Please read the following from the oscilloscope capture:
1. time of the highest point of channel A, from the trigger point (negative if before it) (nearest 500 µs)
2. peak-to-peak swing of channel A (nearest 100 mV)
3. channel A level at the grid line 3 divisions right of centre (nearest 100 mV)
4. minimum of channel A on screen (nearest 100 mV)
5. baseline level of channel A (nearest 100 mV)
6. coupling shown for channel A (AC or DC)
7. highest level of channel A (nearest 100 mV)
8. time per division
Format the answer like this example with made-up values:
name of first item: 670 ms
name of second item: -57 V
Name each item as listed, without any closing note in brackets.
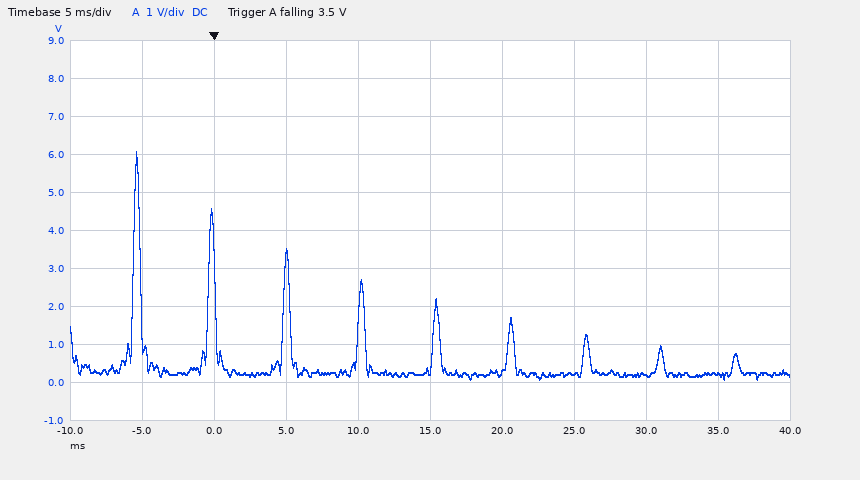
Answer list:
time of the highest point of channel A, from the trigger point (negative if before it): -5.5 ms
peak-to-peak swing of channel A: 6.0 V
channel A level at the grid line 3 divisions right of centre: 200 mV
minimum of channel A on screen: 100 mV
baseline level of channel A: 200 mV
coupling shown for channel A: DC
highest level of channel A: 6.1 V
time per division: 5 ms
